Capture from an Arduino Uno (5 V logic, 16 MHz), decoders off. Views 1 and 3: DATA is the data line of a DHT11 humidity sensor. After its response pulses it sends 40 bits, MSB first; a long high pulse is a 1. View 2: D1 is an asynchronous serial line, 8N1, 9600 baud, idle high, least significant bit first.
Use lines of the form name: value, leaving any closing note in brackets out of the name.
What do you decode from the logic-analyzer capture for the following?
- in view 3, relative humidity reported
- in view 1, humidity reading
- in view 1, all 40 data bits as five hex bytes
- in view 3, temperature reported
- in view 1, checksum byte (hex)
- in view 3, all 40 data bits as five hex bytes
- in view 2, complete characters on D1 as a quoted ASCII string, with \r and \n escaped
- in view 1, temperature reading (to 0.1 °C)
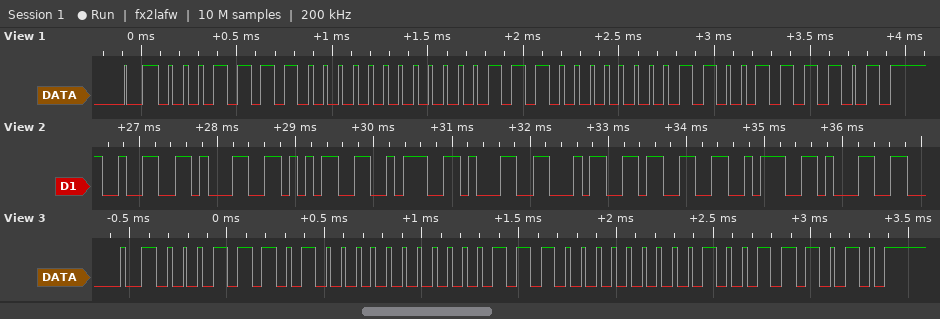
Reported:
in view 3, relative humidity reported: 29 %
in view 1, humidity reading: 30 %
in view 1, all 40 data bits as five hex bytes: 1E 00 1C 03 3D
in view 3, temperature reported: 28.1 °C
in view 1, checksum byte: 0x3D
in view 3, all 40 data bits as five hex bytes: 1D 00 1C 01 3A
in view 2, complete characters on D1 as a quoted ASCII string, with \r and \n escaped: "215:143:1"
in view 1, temperature reading: 28.3 °C
